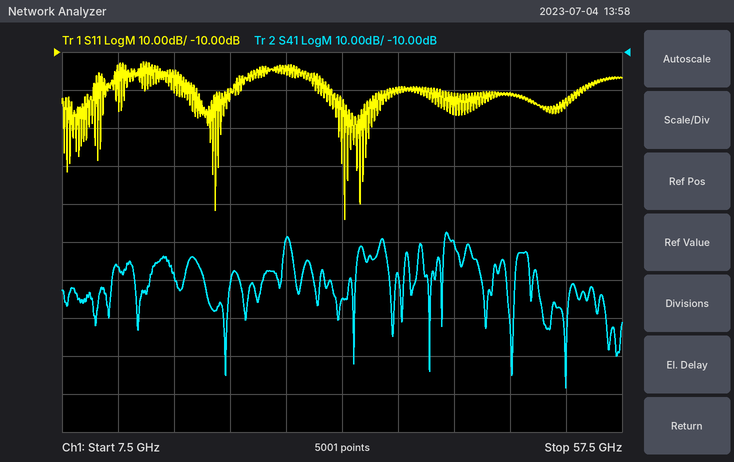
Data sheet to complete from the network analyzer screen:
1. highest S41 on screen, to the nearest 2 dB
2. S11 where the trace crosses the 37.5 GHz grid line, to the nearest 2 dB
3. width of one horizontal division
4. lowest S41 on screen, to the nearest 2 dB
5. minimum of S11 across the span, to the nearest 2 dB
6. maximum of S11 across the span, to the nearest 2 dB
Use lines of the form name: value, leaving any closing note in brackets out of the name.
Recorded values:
highest S41 on screen, to the nearest 2 dB: -58 dB
S11 where the trace crosses the 37.5 GHz grid line, to the nearest 2 dB: -20 dB
width of one horizontal division: 5 GHz
lowest S41 on screen, to the nearest 2 dB: -98 dB
minimum of S11 across the span, to the nearest 2 dB: -54 dB
maximum of S11 across the span, to the nearest 2 dB: -12 dB
